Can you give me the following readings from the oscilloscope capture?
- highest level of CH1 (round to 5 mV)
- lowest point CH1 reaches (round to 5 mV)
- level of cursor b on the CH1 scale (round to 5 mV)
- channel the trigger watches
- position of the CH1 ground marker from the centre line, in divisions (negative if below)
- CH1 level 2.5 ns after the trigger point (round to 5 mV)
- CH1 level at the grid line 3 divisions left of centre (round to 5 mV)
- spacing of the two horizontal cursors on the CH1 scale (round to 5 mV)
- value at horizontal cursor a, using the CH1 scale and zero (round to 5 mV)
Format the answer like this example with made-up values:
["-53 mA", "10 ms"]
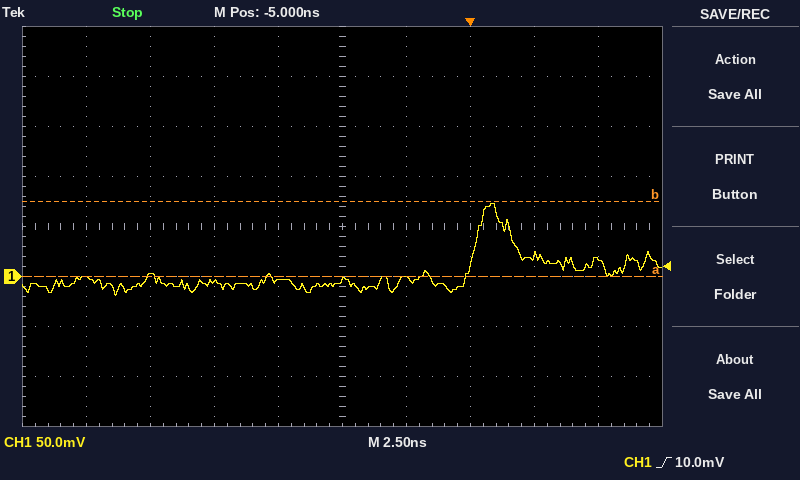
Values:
["75 mV", "-20 mV", "75 mV", "CH1", "-1.0 div", "20 mV", "0 mV", "75 mV", "0 mV"]
